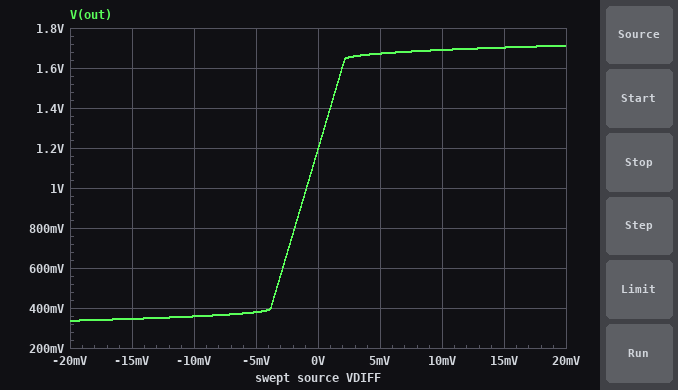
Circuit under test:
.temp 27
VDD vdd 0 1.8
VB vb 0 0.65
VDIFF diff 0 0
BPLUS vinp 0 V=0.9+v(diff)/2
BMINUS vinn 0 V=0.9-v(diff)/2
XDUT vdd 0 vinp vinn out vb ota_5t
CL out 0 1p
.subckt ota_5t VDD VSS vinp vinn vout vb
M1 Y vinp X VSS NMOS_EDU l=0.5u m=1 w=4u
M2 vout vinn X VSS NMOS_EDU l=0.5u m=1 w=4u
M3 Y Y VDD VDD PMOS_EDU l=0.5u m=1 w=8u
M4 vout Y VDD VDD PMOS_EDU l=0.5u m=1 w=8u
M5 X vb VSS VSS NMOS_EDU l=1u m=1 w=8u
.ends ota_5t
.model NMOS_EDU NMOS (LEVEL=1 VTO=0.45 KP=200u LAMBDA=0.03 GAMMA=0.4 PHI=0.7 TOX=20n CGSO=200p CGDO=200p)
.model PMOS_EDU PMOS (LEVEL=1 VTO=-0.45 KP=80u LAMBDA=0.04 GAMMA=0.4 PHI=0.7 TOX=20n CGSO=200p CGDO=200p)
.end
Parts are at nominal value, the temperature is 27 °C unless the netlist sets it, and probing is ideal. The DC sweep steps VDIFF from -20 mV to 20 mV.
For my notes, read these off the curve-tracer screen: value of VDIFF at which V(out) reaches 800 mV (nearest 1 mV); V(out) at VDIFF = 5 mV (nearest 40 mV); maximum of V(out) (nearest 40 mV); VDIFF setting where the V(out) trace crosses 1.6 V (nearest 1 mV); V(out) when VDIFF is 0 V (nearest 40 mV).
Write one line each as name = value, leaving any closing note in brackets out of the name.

value of VDIFF at which V(out) reaches 800 mV = -2 mV
V(out) at VDIFF = 5 mV = 1.68 V
maximum of V(out) = 1.72 V
VDIFF setting where the V(out) trace crosses 1.6 V = 2 mV
V(out) when VDIFF is 0 V = 1.20 V
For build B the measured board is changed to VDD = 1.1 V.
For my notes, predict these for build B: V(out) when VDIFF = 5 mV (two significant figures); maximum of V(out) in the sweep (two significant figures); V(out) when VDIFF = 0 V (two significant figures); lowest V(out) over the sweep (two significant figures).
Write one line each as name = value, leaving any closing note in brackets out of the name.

V(out) when VDIFF = 5 mV = 970 mV
maximum of V(out) in the sweep = 1.0 V
V(out) when VDIFF = 0 V = 490 mV
lowest V(out) over the sweep = 330 mV
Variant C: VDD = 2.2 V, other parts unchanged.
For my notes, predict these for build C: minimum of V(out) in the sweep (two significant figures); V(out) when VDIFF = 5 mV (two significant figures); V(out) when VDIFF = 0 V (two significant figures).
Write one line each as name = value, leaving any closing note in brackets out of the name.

minimum of V(out) in the sweep = 340 mV
V(out) when VDIFF = 5 mV = 2.1 V
V(out) when VDIFF = 0 V = 1.6 V
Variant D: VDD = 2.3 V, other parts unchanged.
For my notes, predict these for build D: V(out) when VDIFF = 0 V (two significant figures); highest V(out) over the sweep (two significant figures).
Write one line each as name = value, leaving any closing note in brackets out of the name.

V(out) when VDIFF = 0 V = 1.7 V
highest V(out) over the sweep = 2.2 V
